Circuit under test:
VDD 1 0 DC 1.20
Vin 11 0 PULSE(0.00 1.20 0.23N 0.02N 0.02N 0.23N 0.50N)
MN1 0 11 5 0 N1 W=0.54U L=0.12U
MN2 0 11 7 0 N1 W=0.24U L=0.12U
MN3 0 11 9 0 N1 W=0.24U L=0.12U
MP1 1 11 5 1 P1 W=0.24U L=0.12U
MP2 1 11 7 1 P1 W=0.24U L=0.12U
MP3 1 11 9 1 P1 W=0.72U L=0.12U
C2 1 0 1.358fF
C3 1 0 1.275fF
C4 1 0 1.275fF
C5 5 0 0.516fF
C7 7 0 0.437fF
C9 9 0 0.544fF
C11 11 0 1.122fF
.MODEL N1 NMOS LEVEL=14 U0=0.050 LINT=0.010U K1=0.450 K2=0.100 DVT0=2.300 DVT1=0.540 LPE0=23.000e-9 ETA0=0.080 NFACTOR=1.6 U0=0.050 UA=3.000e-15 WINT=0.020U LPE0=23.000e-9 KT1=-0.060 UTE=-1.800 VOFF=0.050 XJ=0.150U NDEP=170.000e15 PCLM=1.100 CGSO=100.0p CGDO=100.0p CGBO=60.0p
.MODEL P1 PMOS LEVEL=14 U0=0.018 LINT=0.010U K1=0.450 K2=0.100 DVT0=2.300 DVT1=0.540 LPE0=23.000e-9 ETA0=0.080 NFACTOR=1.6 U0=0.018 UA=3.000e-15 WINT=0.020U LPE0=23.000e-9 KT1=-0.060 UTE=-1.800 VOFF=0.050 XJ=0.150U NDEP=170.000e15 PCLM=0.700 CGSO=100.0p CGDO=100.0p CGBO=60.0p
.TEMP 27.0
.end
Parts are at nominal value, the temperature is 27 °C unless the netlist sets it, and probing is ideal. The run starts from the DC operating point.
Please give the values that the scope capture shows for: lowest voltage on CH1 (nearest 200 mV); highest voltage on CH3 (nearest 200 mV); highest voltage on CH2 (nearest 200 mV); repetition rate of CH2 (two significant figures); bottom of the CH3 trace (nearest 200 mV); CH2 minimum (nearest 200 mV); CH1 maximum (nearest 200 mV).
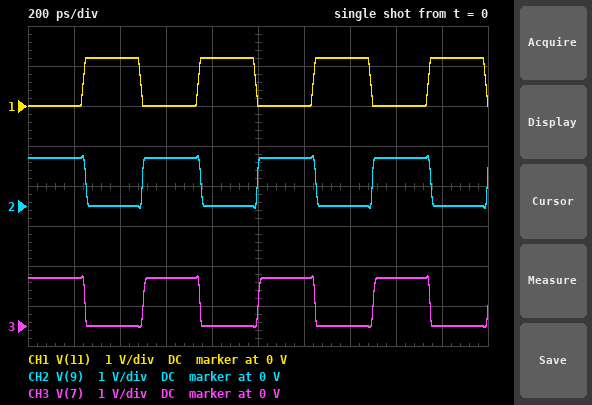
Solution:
0 V
1.2 V
1.2 V
2.0 GHz
0 V
0 V
1.2 V
